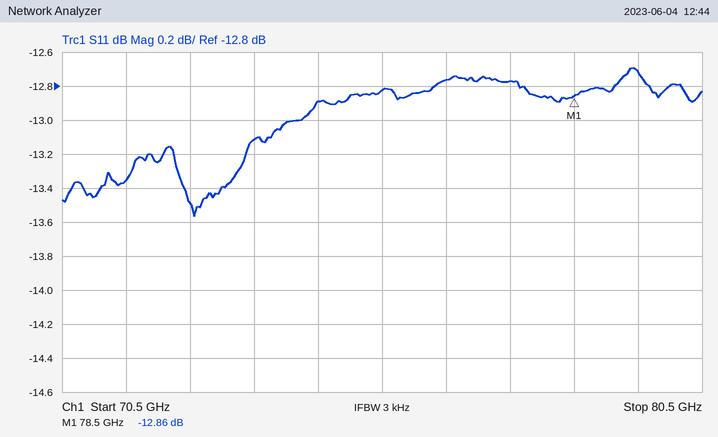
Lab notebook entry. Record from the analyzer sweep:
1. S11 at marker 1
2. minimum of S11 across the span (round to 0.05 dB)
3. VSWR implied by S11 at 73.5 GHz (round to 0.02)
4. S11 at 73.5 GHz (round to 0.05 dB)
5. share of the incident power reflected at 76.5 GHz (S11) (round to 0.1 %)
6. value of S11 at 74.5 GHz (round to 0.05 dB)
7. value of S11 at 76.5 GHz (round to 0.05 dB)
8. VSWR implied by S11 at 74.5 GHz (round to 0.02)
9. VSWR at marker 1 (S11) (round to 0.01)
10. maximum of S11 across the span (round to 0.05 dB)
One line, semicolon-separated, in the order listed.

-12.86 dB; -13.55 dB; 1.56; -13.10 dB; 5.3 %; -12.90 dB; -12.75 dB; 1.58; 1.59; -12.70 dB
